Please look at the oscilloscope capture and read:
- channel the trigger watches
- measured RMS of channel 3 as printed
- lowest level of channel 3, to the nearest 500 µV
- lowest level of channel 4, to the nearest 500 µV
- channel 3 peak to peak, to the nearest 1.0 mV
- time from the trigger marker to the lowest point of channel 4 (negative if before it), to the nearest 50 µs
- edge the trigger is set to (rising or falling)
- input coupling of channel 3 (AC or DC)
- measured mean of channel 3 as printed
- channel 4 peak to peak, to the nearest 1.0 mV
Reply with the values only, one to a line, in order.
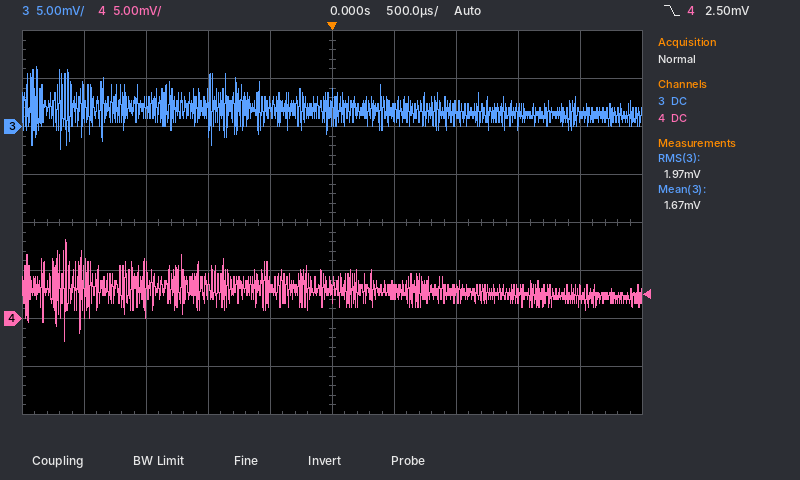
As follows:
channel 4
1.97 mV
-2.5 mV
-2.5 mV
9.0 mV
-2.15 ms
falling
DC
1.67 mV
11.0 mV
